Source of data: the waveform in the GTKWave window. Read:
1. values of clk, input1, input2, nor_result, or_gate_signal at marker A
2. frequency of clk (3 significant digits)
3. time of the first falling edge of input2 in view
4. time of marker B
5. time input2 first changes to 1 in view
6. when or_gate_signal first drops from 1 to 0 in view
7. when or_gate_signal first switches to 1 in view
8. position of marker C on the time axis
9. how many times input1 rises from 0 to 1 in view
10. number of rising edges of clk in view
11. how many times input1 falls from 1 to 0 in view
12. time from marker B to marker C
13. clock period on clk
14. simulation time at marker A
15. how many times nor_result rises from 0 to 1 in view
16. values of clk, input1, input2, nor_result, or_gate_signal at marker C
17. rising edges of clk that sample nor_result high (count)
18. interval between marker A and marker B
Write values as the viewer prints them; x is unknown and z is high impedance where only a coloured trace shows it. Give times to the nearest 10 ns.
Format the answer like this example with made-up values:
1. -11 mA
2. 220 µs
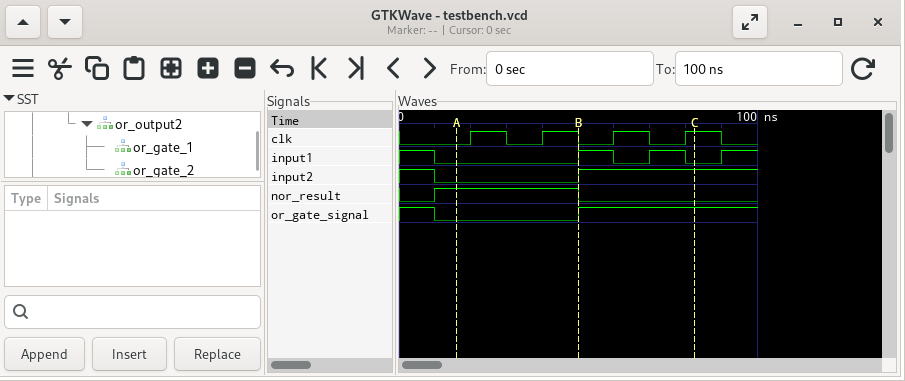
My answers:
1. clk=0, input1=0, input2=0, nor_result=1, or_gate_signal=0
2. 50.0 MHz
3. 10 ns
4. 50 ns
5. 50 ns
6. 10 ns
7. 50 ns
8. 80 ns
9. 3
10. 4
11. 3
12. 30 ns
13. 20 ns
14. 20 ns
15. 1
16. clk=1, input1=0, input2=1, nor_result=0, or_gate_signal=1
17. 2
18. 30 ns
